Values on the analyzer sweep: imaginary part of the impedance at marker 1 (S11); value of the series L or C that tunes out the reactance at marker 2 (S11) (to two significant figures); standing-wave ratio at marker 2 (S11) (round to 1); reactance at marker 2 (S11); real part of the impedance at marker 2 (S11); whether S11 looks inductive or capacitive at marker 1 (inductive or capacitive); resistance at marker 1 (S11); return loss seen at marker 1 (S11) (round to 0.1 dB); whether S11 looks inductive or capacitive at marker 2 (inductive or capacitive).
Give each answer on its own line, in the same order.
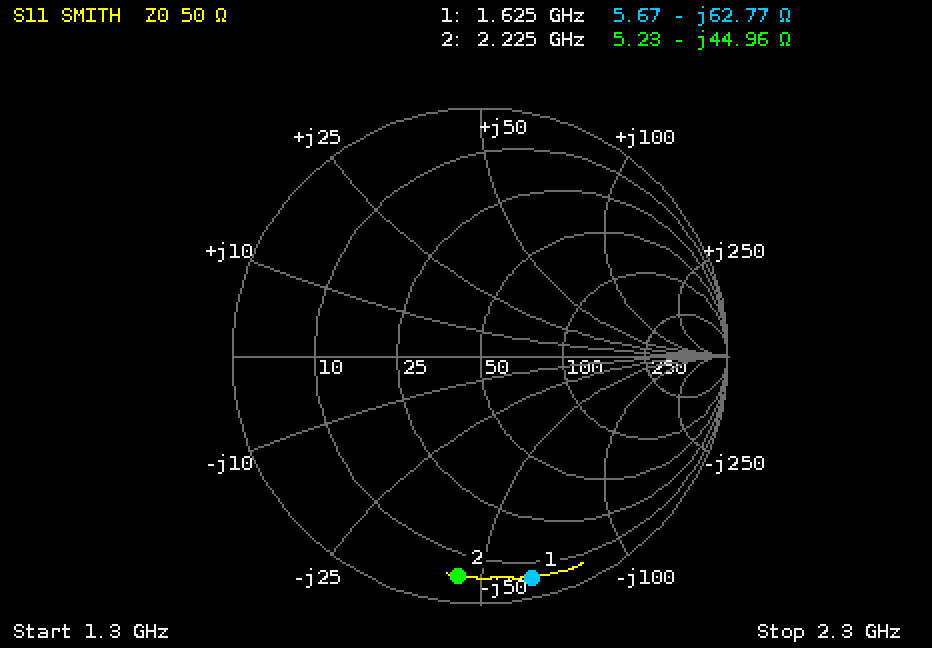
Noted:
-62.77 Ω
3.2 nH
17
-44.96 Ω
5.23 Ω
capacitive
5.67 Ω
0.8 dB
capacitive
